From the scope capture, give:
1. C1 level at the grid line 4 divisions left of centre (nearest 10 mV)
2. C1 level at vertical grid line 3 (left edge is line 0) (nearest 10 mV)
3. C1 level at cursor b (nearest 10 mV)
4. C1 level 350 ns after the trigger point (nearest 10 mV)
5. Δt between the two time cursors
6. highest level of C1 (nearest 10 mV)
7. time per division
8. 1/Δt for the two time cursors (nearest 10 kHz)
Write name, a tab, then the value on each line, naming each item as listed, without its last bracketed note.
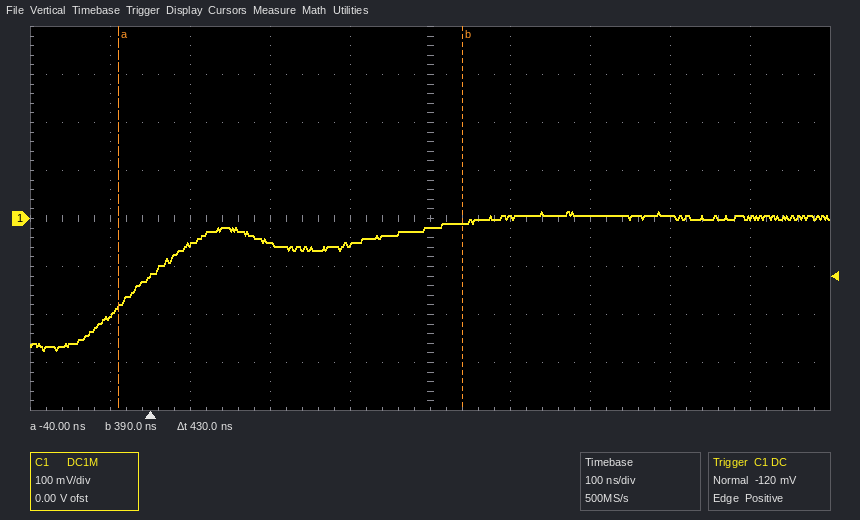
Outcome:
C1 level at the grid line 4 divisions left of centre	-200 mV
C1 level at vertical grid line 3 (left edge is line 0)	-50 mV
C1 level at cursor b	-10 mV
C1 level 350 ns after the trigger point	-20 mV
Δt between the two time cursors	430 ns
highest level of C1	10 mV
time per division	100 ns
1/Δt for the two time cursors	2.33 MHz
